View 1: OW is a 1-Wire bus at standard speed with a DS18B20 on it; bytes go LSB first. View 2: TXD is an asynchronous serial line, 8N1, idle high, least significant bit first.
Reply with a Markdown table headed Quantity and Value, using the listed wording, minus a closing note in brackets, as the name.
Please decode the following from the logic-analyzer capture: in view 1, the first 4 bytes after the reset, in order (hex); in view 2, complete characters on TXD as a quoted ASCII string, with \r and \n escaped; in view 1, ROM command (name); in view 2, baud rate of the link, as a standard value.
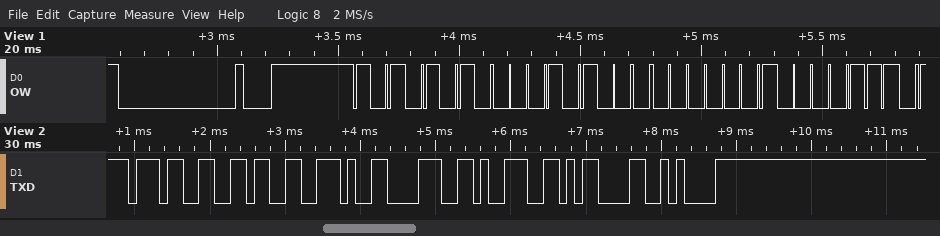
| Quantity | Value |
|---|---|
| in view 1, the first 4 bytes after the reset, in order | 55 28 80 70 |
| in view 2, complete characters on TXD as a quoted ASCII string, with \r and \n escaped | "76.89\r\n" |
| in view 1, ROM command | Match ROM |
| in view 2, baud rate of the link, as a standard value | 9600 baud |
